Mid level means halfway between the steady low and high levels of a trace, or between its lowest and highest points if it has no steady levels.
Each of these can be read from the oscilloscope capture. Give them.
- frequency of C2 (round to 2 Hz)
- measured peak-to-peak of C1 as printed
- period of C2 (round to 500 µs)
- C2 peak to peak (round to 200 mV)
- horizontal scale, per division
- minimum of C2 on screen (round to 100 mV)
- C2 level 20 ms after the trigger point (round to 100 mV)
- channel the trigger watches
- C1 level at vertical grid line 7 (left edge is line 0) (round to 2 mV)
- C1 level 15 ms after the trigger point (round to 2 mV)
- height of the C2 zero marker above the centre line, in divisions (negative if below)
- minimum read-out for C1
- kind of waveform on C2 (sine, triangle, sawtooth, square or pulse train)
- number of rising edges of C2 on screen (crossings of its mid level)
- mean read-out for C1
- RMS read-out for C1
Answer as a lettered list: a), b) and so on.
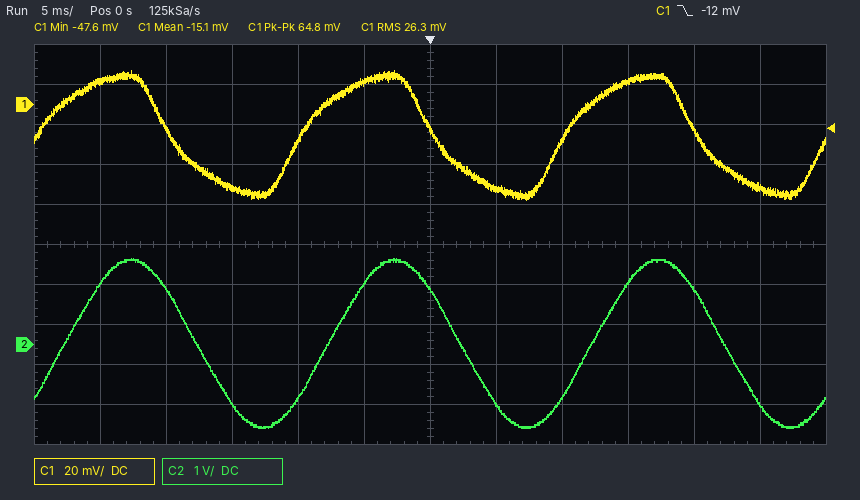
a) 50 Hz
b) 64.8 mV
c) 20.0 ms
d) 4.2 V
e) 5 ms
f) -2.1 V
g) 1.4 V
h) C1
i) -42 mV
j) 12 mV
k) -2.5 div
l) -47.6 mV
m) sine
n) 3
o) -15.1 mV
p) 26.3 mV
